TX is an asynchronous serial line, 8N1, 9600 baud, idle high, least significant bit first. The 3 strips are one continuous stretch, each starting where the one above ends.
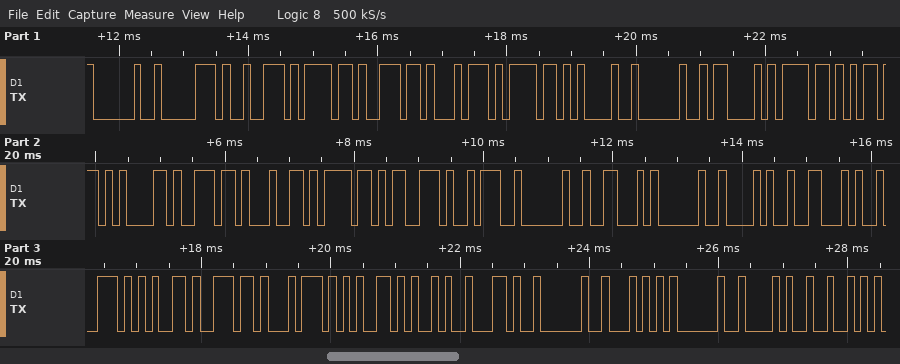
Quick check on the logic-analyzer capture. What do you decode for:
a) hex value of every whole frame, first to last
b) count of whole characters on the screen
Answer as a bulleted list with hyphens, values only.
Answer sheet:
- 20 70 72 6F 6E 74 6F 21 20 43 6F 6D 61 6E 64 6F 73 3A 20 46 20 28 46 72 65 6E 74 65 29 2C 20 54 20 28 52
- 35
